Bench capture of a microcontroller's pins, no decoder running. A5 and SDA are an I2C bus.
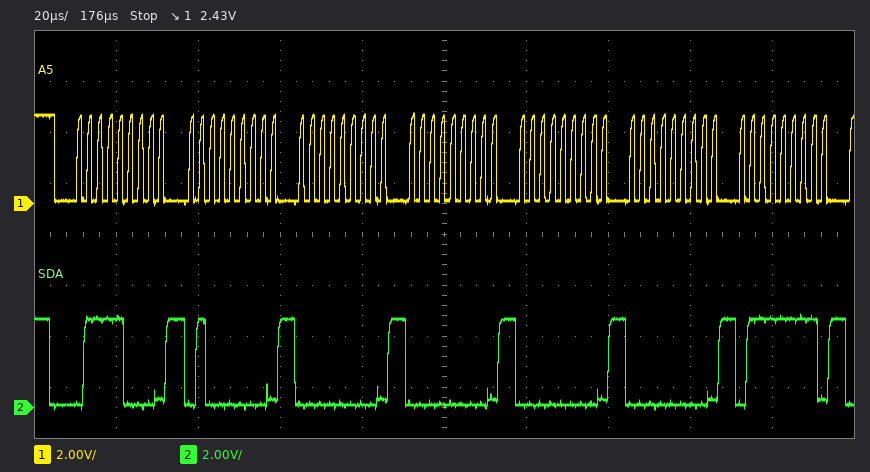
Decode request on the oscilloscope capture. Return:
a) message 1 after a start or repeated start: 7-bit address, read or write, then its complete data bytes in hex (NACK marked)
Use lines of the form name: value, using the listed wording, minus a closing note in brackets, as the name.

message 1 after a start or repeated start: 7-bit address, read or write, then its complete data bytes in hex: 0x3C write: 40 00 00 00 00 7F
